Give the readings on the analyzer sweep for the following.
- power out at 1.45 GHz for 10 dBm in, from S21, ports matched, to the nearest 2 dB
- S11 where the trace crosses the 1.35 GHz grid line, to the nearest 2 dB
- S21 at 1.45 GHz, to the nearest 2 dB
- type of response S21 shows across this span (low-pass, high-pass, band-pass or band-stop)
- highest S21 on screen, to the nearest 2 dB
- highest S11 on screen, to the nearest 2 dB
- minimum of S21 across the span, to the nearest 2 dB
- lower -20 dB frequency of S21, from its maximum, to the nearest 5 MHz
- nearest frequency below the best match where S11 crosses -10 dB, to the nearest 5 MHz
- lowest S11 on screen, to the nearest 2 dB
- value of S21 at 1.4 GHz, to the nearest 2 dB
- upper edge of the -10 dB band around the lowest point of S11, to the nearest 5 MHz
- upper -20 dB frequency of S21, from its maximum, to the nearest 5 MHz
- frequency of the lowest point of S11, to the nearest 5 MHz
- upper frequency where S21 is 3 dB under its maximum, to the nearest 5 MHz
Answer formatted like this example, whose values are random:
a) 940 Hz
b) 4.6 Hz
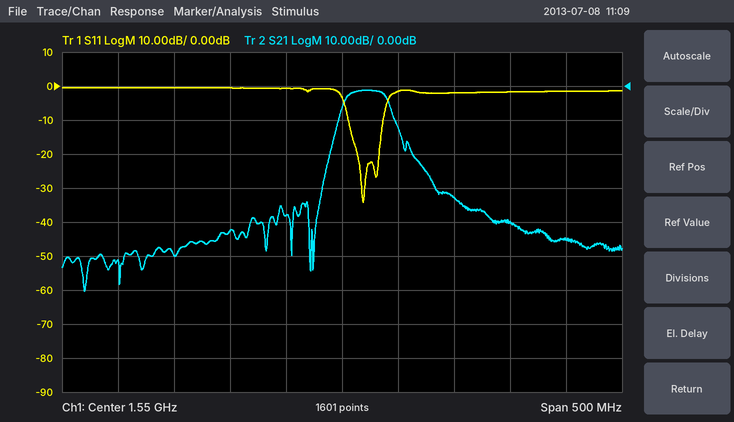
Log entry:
a) -32 dBm
b) 0 dB
c) -42 dB
d) band-pass
e) -2 dB
f) 0 dB
g) -60 dB
h) 1.540 GHz
i) 1.555 GHz
j) -34 dB
k) -50 dB
l) 1.585 GHz
m) 1.615 GHz
n) 1.570 GHz
o) 1.590 GHz
